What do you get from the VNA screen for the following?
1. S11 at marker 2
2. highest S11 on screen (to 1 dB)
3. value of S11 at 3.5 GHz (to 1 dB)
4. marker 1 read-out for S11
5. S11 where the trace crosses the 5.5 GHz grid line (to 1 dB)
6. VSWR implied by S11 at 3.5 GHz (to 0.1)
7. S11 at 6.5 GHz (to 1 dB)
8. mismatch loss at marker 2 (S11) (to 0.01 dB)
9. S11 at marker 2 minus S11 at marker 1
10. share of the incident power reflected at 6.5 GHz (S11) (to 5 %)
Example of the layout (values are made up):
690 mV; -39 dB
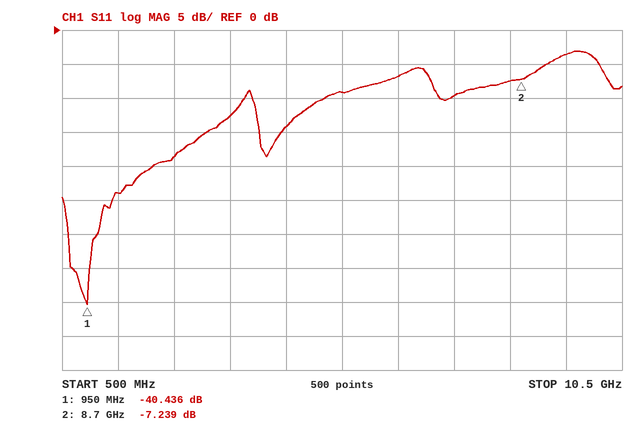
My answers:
-7.239 dB; -3 dB; -13 dB; -40.436 dB; -9 dB; 1.6; -7 dB; 0.91 dB; 33.197 dB; 20 %
